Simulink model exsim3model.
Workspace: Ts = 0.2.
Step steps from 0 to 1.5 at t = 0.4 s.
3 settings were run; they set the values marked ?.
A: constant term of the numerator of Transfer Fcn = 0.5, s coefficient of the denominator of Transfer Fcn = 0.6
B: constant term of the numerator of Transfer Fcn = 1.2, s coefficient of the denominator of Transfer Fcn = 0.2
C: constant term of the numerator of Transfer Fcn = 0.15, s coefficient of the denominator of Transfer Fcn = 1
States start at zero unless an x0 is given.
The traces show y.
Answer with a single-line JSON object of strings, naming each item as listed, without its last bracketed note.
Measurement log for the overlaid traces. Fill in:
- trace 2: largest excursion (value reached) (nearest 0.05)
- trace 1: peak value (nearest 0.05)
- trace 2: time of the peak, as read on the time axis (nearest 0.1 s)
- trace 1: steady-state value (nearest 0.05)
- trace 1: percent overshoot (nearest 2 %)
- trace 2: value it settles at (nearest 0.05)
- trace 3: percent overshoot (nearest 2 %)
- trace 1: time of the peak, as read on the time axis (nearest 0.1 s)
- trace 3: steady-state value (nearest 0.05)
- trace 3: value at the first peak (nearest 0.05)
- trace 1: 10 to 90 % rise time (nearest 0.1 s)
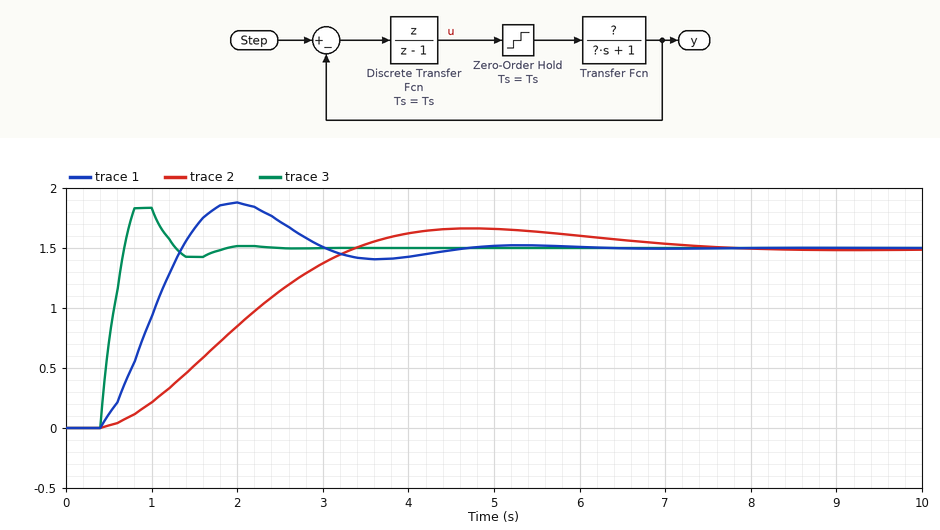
{"trace 2: largest excursion (value reached)": "1.65", "trace 1: peak value": "1.90", "trace 2: time of the peak, as read on the time axis": "4.8 s", "trace 1: steady-state value": "1.50", "trace 1: percent overshoot": "26 %", "trace 2: value it settles at": "1.50", "trace 3: percent overshoot": "22 %", "trace 1: time of the peak, as read on the time axis": "2.0 s", "trace 3: steady-state value": "1.50", "trace 3: value at the first peak": "1.85", "trace 1: 10 to 90 % rise time": "0.7 s"}
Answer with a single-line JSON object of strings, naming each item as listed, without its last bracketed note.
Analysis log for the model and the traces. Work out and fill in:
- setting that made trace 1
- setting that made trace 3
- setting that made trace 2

{"setting that made trace 1": "A", "setting that made trace 3": "B", "setting that made trace 2": "C"}
